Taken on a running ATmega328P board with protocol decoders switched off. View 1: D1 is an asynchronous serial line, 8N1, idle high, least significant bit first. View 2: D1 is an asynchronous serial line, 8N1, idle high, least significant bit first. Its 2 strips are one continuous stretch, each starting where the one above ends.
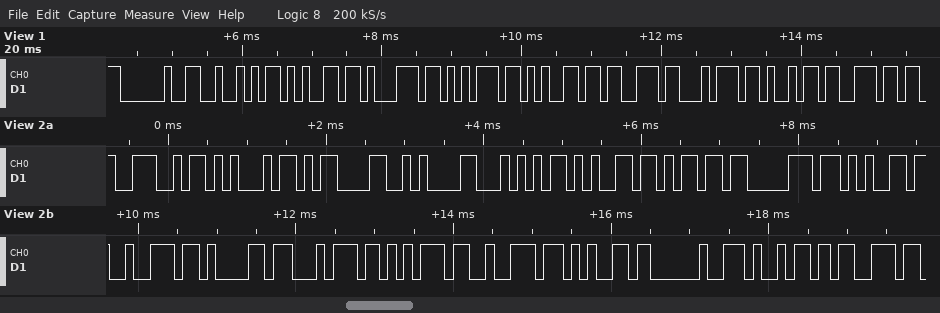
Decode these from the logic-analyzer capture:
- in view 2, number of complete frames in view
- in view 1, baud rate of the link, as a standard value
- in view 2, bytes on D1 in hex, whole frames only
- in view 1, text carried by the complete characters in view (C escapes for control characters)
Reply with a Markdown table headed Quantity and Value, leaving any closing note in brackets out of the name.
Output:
| Quantity | Value |
|---|---|
| in view 2, number of complete frames in view | 18 |
| in view 1, baud rate of the link, as a standard value | 9600 baud |
| in view 2, bytes on D1 in hex, whole frames only | 0x4E 0x45 0x0D 0x0A 0x54 0x65 0x6D 0x70 0x65 0x72 0x61 0x74 0x75 0x72 0x65 0x20 0x69 0x73 |
| in view 1, text carried by the complete characters in view | " Requestin" |
